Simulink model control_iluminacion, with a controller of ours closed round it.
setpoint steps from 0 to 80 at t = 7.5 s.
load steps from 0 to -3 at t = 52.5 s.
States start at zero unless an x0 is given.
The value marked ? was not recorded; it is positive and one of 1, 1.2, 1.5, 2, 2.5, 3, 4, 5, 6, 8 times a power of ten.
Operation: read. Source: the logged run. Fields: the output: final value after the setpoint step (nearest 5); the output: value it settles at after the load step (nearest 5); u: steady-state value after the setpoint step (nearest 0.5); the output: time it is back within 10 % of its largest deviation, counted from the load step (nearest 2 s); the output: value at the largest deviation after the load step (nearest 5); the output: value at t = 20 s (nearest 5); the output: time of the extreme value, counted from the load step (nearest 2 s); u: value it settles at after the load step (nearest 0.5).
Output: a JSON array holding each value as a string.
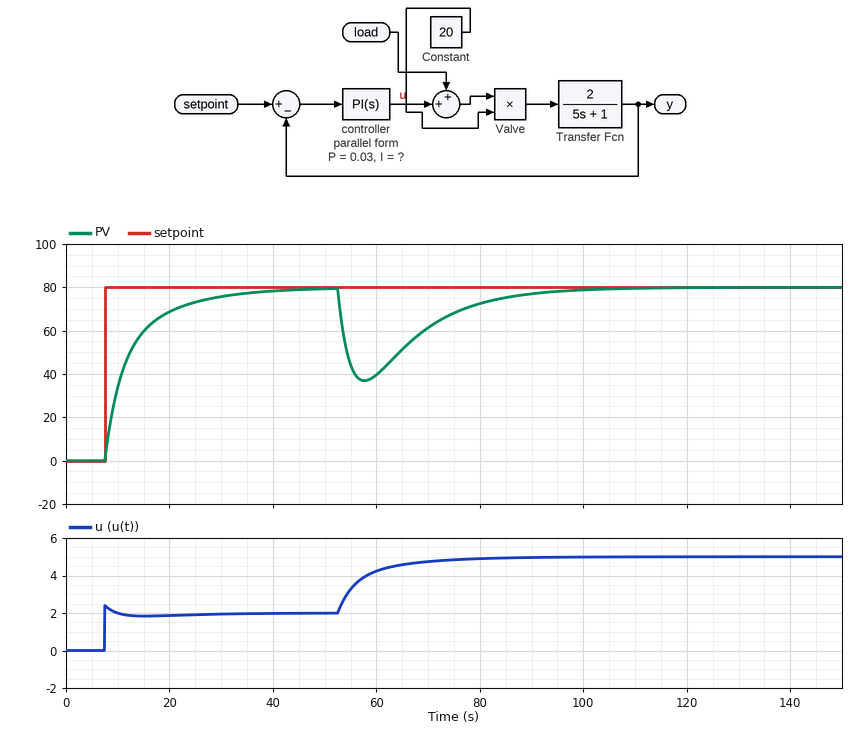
["80", "80", "2.0", "34 s", "35", "70", "6 s", "5.0"]
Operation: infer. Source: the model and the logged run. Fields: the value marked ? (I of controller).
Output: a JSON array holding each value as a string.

["0.004"]
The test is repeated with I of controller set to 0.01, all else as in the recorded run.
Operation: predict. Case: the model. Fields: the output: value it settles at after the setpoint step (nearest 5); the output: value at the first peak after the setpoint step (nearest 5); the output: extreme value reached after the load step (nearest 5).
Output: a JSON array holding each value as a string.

["80", "85", "45"]
